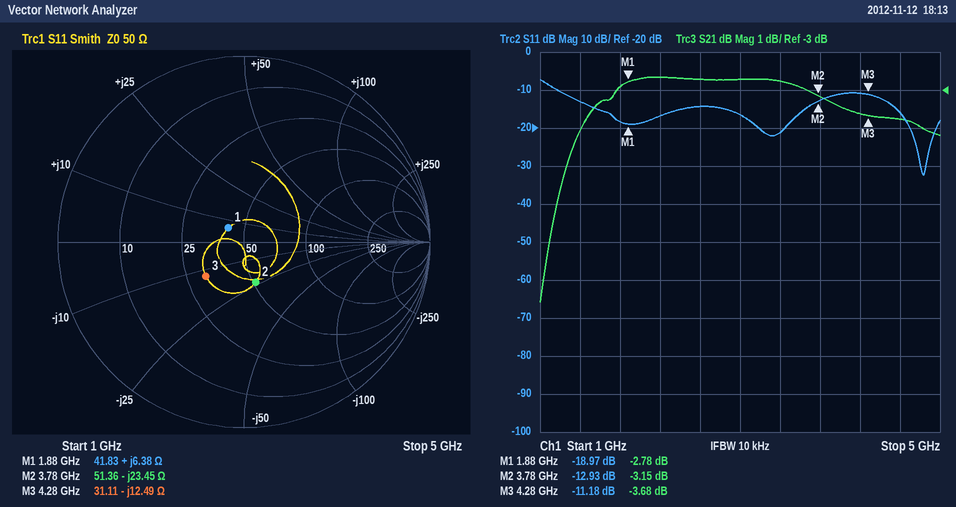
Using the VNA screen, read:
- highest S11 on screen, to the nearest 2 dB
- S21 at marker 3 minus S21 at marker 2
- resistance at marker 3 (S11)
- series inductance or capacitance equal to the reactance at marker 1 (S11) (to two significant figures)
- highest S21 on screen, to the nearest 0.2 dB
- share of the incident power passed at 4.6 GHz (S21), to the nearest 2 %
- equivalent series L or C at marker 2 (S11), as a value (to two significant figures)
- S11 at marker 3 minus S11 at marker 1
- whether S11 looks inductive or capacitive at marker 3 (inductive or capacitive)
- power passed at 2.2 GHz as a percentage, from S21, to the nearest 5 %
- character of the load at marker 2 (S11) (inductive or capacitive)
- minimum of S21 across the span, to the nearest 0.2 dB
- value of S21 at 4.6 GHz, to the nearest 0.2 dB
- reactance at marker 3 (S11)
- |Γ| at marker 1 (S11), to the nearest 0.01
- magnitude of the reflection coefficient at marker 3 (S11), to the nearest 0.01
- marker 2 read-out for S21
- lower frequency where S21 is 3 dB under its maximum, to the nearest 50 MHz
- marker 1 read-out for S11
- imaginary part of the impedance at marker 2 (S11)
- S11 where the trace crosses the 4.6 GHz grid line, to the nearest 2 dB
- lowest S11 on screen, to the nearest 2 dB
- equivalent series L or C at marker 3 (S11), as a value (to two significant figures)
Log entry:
-8 dB
-0.53 dB
31.11 Ω
540 pH
-2.6 dB
42 %
1.8 pF
7.79 dB
capacitive
55 %
capacitive
-8.6 dB
-3.8 dB
-12.49 Ω
0.11
0.28
-3.15 dB
1.20 GHz
-18.97 dB
-23.45 Ω
-16 dB
-32 dB
3.0 pF
